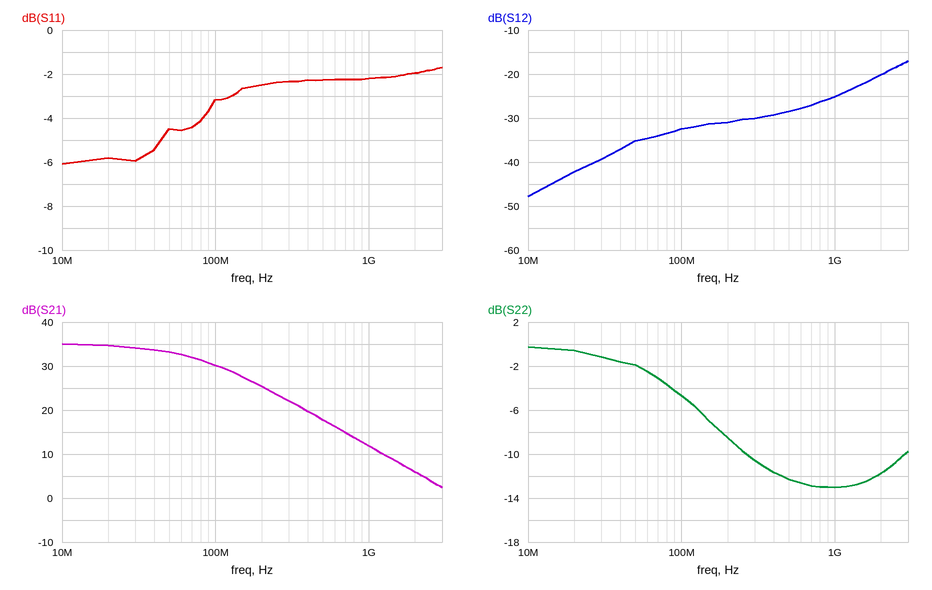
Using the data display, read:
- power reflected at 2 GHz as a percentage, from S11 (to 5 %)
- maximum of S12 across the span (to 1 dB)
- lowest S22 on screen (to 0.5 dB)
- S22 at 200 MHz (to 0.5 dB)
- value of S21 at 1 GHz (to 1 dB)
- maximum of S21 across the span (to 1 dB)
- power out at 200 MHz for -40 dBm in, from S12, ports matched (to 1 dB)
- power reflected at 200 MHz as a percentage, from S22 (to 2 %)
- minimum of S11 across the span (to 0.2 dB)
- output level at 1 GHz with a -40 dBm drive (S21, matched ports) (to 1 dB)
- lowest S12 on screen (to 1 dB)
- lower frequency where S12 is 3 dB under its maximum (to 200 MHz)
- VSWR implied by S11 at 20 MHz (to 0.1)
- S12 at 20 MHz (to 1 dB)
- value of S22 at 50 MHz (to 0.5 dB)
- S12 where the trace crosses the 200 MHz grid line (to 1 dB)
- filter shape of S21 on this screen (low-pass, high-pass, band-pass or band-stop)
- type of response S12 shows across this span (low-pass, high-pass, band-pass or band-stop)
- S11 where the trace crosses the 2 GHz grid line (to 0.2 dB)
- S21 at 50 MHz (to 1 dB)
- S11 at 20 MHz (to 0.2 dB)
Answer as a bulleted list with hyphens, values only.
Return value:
- 65 %
- -17 dB
- -13.0 dB
- -8.5 dB
- 12 dB
- 35 dB
- -71 dBm
- 14 %
- -6.0 dB
- -28 dBm
- -48 dB
- 2.0 GHz
- 3.1
- -42 dB
- -2.0 dB
- -31 dB
- low-pass
- high-pass
- -2.0 dB
- 33 dB
- -5.8 dB
